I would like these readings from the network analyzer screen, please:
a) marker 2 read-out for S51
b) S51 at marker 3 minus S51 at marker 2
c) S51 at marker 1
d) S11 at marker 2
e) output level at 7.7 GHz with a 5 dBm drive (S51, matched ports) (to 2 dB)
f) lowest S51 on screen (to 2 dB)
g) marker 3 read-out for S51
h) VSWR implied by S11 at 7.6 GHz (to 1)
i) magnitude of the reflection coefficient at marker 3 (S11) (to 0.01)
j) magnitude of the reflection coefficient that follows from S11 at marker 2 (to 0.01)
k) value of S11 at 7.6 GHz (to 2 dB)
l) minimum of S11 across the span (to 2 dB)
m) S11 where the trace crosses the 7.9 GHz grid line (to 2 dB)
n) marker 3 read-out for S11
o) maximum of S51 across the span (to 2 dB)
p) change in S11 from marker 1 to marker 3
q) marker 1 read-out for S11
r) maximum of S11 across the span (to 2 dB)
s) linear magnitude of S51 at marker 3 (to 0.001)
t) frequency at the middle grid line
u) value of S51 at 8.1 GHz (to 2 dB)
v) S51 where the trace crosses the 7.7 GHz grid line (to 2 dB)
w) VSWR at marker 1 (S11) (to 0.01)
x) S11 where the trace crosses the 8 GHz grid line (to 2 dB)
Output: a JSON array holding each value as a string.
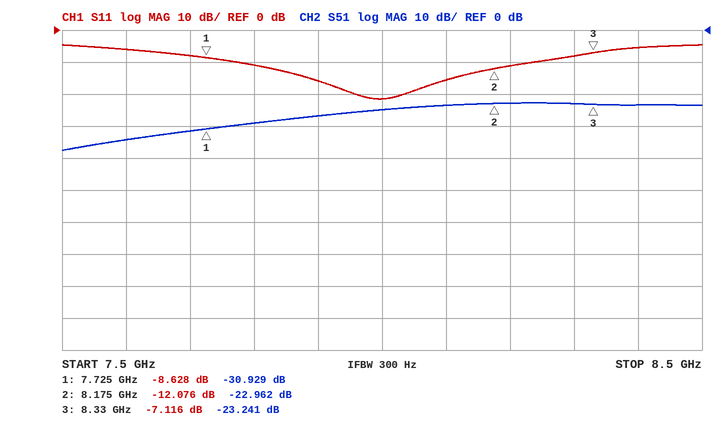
["-22.962 dB", "-0.279 dB", "-30.929 dB", "-12.076 dB", "-26 dBm", "-38 dB", "-23.241 dB", "3", "0.44", "0.25", "-6 dB", "-22 dB", "-16 dB", "-7.116 dB", "-22 dB", "1.512 dB", "-8.628 dB", "-4 dB", "0.069", "8 GHz", "-24 dB", "-32 dB", "2.18", "-22 dB"]
